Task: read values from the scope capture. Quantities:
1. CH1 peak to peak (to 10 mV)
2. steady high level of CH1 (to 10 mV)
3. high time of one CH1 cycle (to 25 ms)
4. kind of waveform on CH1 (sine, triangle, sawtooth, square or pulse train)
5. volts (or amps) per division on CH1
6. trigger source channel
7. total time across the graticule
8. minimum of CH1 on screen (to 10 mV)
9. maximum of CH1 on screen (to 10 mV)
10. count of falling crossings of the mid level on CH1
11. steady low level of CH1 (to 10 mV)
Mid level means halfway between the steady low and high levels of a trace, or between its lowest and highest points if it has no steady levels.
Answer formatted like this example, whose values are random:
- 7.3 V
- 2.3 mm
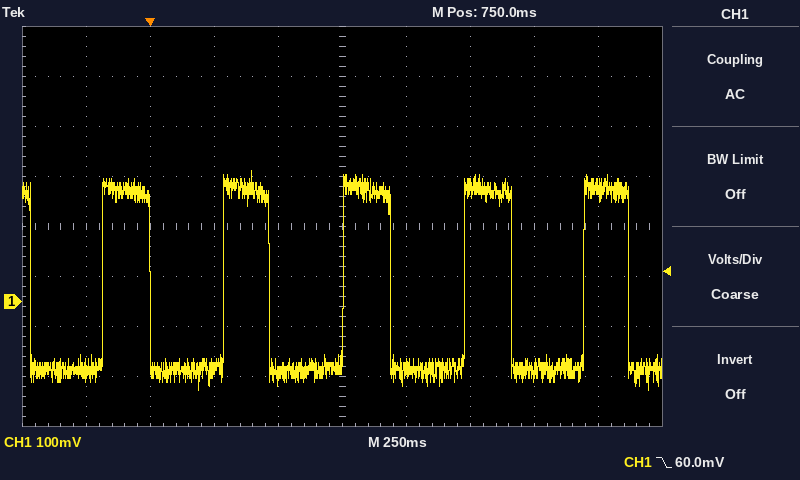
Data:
- 440 mV
- 220 mV
- 175 ms
- pulse train
- 100 mV
- CH1
- 2.5 s
- -180 mV
- 260 mV
- 6
- -140 mV
